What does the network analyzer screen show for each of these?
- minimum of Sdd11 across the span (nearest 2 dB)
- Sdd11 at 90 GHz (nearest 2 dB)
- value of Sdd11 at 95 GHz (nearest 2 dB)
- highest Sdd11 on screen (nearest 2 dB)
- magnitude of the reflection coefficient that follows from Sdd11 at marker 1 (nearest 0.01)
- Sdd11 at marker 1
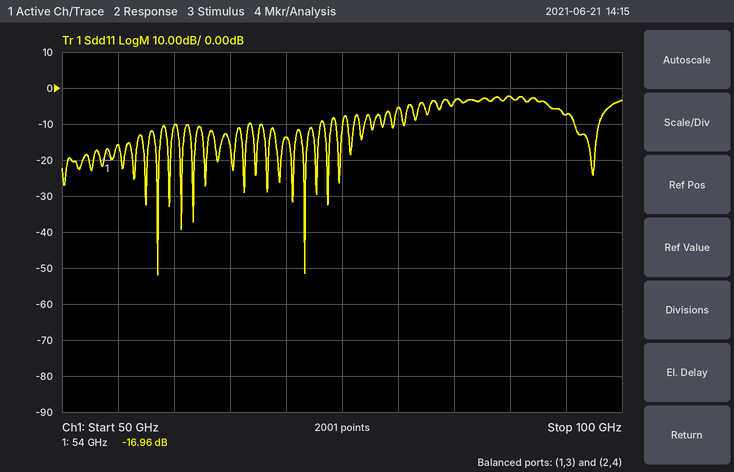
-52 dB
-2 dB
-8 dB
-2 dB
0.14
-16.96 dB
